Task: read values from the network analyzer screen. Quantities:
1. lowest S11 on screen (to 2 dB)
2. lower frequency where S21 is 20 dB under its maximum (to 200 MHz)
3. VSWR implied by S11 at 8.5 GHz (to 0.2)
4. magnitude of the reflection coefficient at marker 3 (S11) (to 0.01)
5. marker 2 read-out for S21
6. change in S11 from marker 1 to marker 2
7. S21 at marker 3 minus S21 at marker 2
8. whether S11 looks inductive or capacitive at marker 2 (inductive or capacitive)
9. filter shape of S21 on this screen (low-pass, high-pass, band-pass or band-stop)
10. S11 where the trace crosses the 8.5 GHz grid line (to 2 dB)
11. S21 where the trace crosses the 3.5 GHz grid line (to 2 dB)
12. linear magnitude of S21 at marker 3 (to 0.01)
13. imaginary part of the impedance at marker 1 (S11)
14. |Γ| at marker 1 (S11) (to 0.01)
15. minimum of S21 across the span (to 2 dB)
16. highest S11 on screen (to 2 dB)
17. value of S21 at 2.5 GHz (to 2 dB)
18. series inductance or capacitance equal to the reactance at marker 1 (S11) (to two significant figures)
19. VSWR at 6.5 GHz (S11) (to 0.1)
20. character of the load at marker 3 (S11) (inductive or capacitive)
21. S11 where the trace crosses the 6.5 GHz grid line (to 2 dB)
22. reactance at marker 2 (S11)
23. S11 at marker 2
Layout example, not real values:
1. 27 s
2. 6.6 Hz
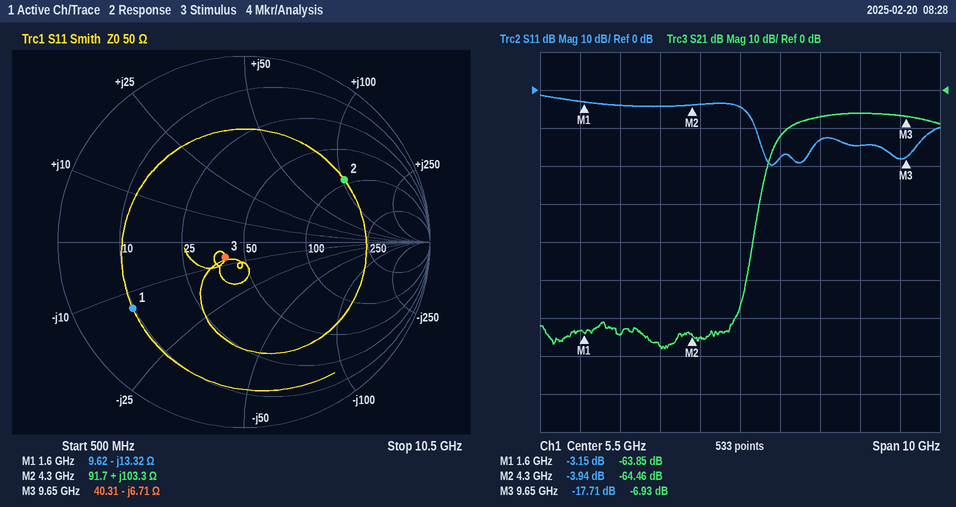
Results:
1. -20 dB
2. 6.0 GHz
3. 1.4
4. 0.13
5. -64.46 dB
6. -0.79 dB
7. 57.53 dB
8. inductive
9. high-pass
10. -14 dB
11. -68 dB
12. 0.45
13. -13.32 Ω
14. 0.70
15. -68 dB
16. -2 dB
17. -64 dB
18. 7.5 pF
19. 1.3
20. capacitive
21. -18 dB
22. +103.3 Ω
23. -3.94 dB
